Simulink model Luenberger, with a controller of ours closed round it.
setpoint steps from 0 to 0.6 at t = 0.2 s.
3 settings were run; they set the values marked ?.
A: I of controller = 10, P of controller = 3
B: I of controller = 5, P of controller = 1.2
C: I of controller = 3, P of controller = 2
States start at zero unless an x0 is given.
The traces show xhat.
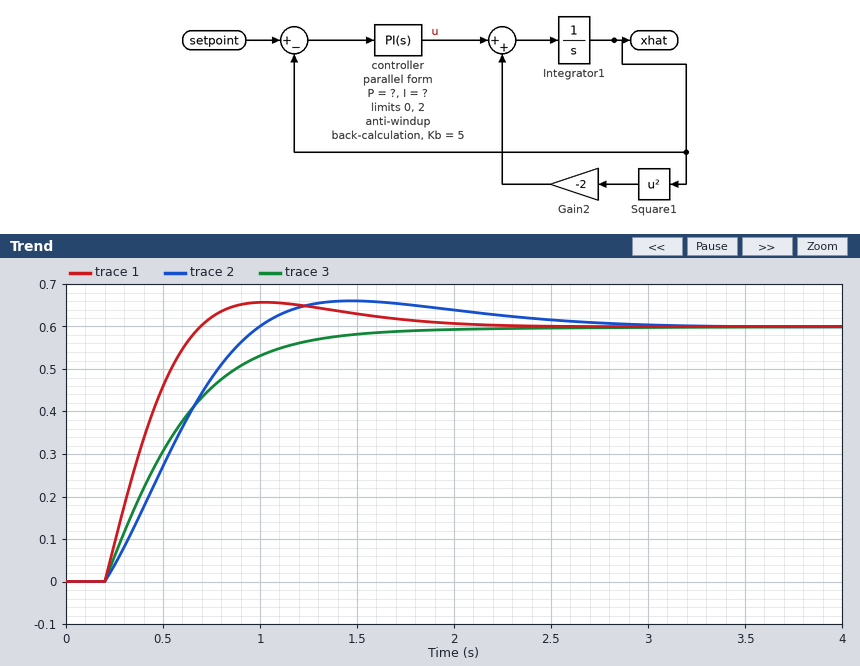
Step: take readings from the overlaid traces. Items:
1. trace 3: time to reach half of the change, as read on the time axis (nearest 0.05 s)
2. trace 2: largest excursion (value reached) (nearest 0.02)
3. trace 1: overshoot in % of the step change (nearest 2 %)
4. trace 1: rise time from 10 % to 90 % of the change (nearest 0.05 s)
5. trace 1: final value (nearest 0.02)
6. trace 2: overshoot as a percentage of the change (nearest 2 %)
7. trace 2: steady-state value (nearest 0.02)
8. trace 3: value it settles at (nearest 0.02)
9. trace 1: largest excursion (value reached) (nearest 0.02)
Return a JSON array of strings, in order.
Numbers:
["0.50 s", "0.66", "10 %", "0.35 s", "0.60", "10 %", "0.60", "0.60", "0.66"]
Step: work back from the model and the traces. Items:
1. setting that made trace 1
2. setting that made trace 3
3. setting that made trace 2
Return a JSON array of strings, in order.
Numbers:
["A", "C", "B"]
